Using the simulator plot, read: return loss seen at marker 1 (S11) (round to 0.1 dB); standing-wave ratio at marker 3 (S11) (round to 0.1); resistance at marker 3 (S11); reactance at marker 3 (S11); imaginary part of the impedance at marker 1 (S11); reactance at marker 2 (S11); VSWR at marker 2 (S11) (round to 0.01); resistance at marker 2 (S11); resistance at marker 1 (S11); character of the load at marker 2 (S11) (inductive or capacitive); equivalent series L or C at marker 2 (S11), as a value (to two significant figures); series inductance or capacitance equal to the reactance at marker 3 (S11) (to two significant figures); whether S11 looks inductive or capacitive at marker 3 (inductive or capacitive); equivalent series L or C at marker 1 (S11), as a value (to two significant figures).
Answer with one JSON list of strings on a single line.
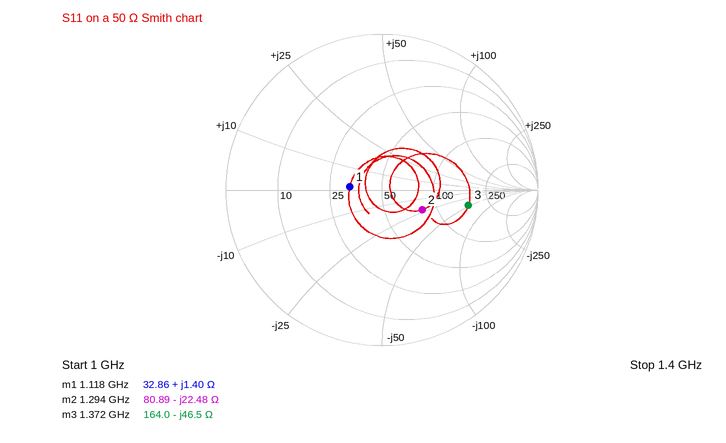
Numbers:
["13.7 dB", "3.6", "164.0 Ω", "-46.5 Ω", "+1.40 Ω", "-22.48 Ω", "1.81", "80.89 Ω", "32.86 Ω", "capacitive", "5.5 pF", "2.5 pF", "capacitive", "200 pH"]
